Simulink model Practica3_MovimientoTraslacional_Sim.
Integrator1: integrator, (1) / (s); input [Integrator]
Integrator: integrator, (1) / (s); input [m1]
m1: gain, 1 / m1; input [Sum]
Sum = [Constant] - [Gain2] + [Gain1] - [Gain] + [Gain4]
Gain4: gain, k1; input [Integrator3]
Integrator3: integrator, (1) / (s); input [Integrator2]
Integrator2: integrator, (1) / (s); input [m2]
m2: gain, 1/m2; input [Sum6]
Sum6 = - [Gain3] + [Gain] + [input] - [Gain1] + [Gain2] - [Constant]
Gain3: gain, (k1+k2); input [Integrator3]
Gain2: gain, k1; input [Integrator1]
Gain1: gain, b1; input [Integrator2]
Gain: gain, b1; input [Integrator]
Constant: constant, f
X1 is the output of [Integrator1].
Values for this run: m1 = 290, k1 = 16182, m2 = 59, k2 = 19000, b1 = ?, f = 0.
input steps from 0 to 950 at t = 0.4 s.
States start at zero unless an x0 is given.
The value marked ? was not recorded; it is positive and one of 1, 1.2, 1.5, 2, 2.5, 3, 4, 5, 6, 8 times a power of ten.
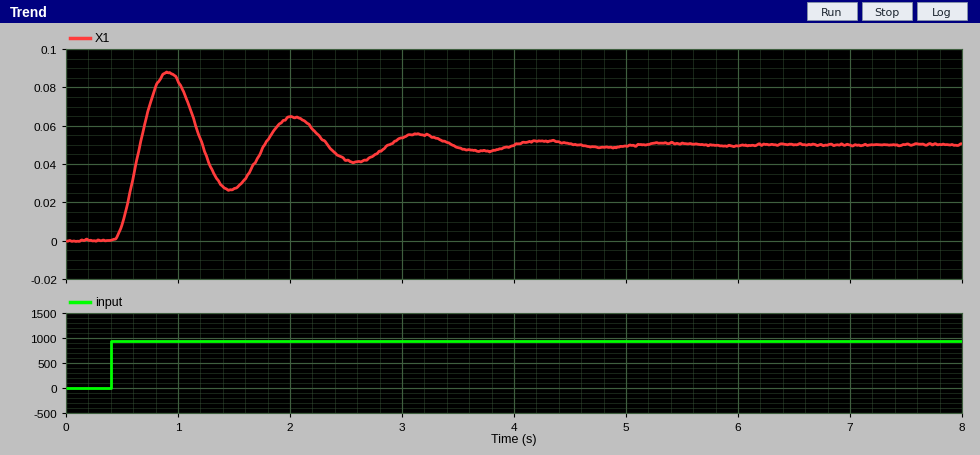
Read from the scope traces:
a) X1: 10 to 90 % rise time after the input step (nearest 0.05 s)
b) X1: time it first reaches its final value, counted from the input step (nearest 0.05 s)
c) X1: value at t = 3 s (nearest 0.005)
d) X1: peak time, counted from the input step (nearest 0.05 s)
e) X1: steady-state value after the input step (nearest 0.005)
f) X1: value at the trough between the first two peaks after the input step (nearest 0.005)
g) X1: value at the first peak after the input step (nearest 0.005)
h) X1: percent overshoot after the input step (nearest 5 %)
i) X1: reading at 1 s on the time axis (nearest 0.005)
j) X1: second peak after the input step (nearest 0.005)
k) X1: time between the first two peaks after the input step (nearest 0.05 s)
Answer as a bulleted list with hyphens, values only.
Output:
- 0.15 s
- 0.25 s
- 0.055
- 0.50 s
- 0.050
- 0.025
- 0.090
- 75 %
- 0.085
- 0.065
- 1.10 s
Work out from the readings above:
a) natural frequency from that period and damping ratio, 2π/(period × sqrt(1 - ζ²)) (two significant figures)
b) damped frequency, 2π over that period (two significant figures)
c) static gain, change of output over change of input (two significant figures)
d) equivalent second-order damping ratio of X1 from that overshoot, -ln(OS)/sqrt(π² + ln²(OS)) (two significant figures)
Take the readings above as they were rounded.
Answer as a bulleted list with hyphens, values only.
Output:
- 5.7 rad/s
- 5.7 rad/s
- 0.000053
- 0.091
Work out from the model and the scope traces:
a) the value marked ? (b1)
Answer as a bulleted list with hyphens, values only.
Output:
- 2000
